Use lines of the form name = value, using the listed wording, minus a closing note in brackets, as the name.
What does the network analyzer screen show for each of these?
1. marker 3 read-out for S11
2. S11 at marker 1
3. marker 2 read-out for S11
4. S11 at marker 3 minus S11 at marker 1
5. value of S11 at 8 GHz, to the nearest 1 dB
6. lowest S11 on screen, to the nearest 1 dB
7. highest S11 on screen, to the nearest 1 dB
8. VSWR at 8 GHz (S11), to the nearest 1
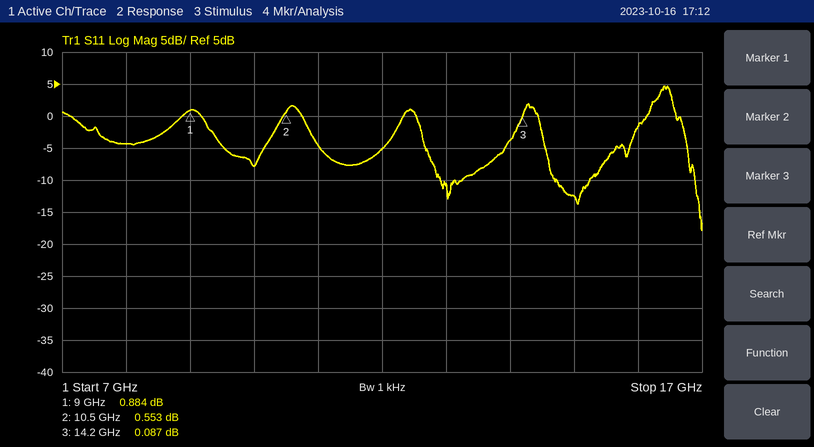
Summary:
marker 3 read-out for S11 = 0.087 dB
S11 at marker 1 = 0.884 dB
marker 2 read-out for S11 = 0.553 dB
S11 at marker 3 minus S11 at marker 1 = -0.797 dB
value of S11 at 8 GHz, to the nearest 1 dB = -4 dB
lowest S11 on screen, to the nearest 1 dB = -18 dB
highest S11 on screen, to the nearest 1 dB = 5 dB
VSWR at 8 GHz (S11), to the nearest 1 = 4
